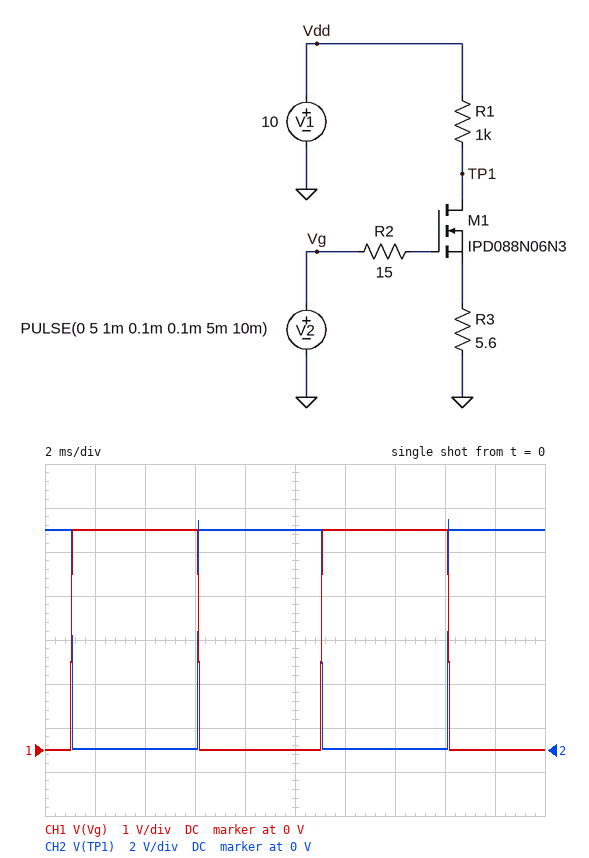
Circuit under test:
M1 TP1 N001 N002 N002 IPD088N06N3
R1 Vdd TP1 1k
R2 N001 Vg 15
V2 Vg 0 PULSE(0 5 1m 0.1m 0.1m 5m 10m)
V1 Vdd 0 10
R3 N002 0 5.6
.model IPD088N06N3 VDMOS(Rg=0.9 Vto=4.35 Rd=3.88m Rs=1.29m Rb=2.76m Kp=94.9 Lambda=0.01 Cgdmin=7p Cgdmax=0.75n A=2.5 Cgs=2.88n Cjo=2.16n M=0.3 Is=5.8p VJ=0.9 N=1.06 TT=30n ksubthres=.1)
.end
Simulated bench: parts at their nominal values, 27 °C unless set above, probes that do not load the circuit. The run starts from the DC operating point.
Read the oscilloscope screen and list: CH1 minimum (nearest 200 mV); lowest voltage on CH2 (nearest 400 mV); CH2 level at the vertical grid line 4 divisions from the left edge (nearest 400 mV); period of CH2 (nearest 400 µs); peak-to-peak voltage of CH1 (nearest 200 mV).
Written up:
0 V
0 V
10.0 V
10.0 ms
5.0 V
